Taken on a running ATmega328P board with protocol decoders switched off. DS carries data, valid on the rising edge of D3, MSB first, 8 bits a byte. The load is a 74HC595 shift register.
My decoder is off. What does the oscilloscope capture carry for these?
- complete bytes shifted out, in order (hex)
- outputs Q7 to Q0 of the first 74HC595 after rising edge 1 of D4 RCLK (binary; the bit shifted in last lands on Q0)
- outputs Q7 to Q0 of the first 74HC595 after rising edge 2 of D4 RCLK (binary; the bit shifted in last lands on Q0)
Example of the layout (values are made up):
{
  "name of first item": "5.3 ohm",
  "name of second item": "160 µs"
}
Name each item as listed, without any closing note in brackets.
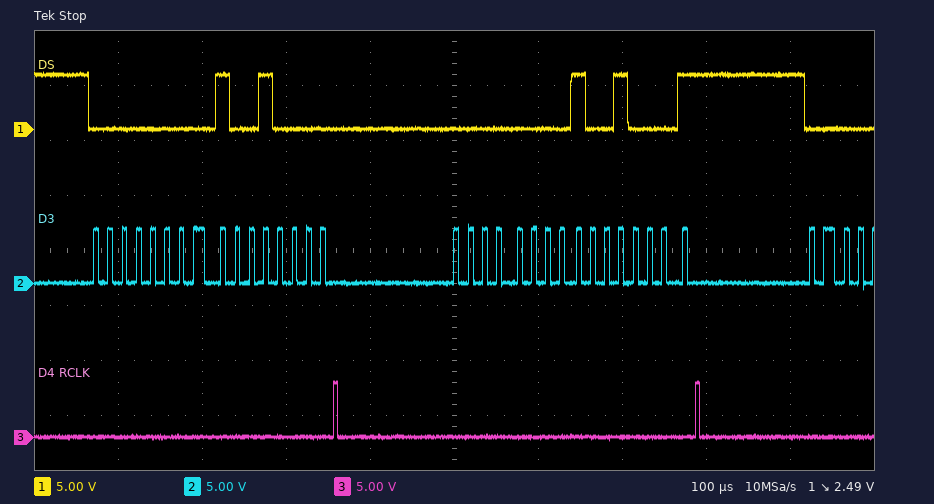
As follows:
{
  "complete bytes shifted out, in order": "0x00 0x90 0x00 0x91",
  "outputs Q7 to Q0 of the first 74HC595 after rising edge 1 of D4 RCLK": "10010000",
  "outputs Q7 to Q0 of the first 74HC595 after rising edge 2 of D4 RCLK": "10010001"
}
